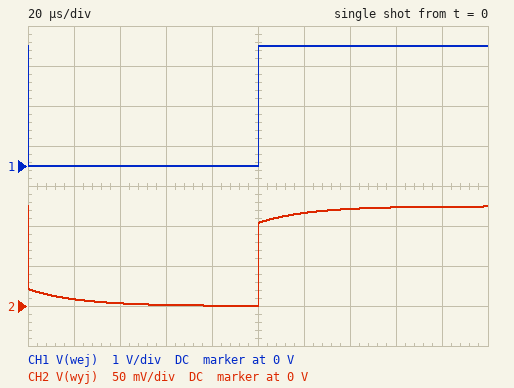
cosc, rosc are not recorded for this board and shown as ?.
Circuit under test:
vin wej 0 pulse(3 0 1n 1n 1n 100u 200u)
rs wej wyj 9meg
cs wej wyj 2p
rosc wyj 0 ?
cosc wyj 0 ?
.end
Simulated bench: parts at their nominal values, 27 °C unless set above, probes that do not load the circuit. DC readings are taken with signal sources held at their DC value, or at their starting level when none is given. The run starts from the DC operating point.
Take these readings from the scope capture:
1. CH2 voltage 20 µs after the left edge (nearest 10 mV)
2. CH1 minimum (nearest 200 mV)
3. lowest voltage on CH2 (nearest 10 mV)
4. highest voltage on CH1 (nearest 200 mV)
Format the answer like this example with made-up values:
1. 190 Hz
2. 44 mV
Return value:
1. 10 mV
2. 0 V
3. 0 V
4. 3.0 V
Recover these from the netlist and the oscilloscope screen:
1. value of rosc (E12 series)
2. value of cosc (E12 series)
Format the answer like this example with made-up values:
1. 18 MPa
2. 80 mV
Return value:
1. 390 kΩ
2. 56 pF
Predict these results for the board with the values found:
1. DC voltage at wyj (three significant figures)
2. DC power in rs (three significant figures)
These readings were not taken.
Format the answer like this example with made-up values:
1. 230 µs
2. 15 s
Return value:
1. 125 mV
2. 919 nW
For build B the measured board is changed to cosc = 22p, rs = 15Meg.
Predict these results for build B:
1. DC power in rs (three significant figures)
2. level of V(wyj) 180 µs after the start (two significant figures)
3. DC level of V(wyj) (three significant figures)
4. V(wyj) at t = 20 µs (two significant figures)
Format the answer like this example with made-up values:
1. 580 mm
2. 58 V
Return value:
1. 570 nW
2. 76 mV
3. 76.0 mV
4. -19 mV
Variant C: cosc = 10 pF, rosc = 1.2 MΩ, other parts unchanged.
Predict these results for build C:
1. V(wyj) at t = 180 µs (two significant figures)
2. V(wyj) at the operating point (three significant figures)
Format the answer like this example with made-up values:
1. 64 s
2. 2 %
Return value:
1. 350 mV
2. 353 mV
